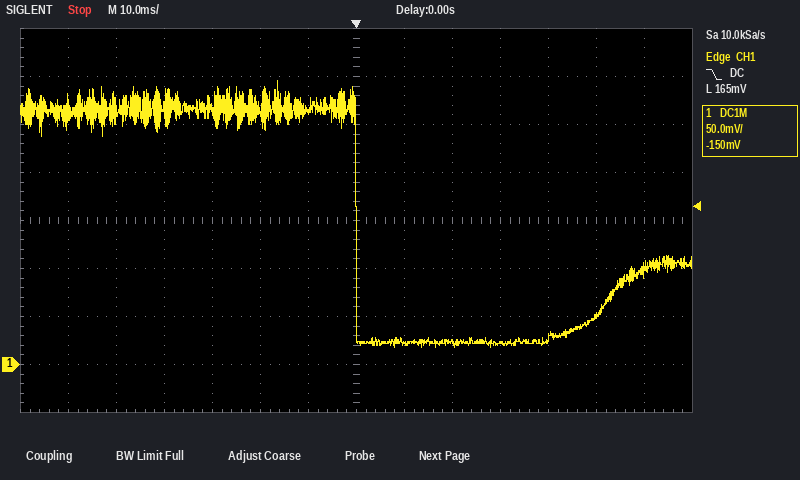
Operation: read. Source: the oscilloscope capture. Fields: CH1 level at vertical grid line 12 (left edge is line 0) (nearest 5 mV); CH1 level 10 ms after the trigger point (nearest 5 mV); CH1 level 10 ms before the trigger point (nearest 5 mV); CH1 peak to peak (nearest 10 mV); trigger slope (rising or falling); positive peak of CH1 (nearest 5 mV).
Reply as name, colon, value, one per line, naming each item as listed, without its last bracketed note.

CH1 level at vertical grid line 12 (left edge is line 0): 50 mV
CH1 level 10 ms after the trigger point: 20 mV
CH1 level 10 ms before the trigger point: 265 mV
CH1 peak to peak: 280 mV
trigger slope: falling
positive peak of CH1: 295 mV
